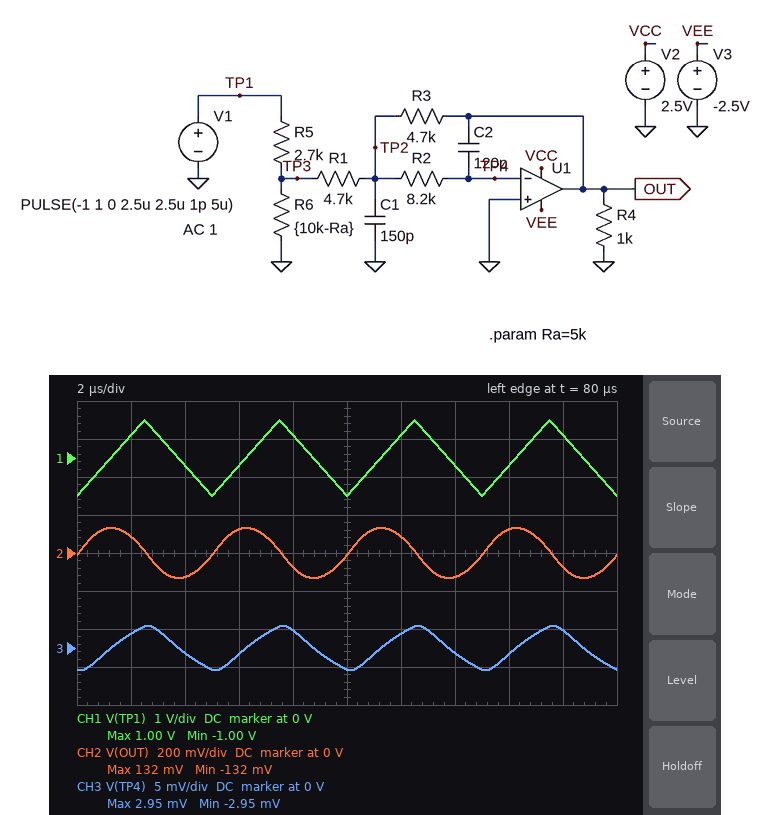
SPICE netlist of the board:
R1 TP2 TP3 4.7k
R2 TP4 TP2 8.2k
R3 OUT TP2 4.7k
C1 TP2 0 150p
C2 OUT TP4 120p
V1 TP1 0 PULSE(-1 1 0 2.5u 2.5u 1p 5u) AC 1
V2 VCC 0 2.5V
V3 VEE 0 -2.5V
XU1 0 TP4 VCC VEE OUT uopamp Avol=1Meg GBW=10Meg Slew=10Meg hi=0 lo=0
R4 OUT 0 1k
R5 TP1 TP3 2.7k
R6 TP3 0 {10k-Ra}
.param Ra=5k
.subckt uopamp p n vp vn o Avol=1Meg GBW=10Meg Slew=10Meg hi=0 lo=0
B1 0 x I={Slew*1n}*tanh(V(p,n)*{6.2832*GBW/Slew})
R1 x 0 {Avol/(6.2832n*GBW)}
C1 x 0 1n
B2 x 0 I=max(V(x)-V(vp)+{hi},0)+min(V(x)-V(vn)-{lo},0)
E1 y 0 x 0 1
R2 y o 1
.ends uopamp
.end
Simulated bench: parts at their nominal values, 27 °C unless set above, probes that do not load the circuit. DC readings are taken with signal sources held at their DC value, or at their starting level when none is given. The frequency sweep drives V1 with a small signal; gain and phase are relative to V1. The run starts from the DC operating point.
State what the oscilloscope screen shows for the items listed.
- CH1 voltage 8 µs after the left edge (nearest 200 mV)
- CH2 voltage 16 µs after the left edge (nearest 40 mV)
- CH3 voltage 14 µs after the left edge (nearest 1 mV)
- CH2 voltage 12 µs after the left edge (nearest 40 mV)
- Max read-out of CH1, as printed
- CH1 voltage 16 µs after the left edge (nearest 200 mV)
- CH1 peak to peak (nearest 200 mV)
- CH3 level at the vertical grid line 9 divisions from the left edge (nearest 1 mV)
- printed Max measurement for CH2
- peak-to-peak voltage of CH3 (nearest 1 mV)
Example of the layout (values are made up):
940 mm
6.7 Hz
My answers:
600 mV
120 mV
-1 mV
80 mV
1.00 V
-200 mV
2.0 V
2 mV
132 mV
6 mV
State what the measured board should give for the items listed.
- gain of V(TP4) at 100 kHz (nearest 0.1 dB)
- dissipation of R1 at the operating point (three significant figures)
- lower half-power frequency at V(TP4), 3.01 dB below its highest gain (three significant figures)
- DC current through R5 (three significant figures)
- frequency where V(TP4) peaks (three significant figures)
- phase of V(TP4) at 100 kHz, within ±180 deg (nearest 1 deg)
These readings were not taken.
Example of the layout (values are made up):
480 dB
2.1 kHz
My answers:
-50.6 dB
47.6 µW
62.3 kHz
195 µA
189 kHz
26 deg
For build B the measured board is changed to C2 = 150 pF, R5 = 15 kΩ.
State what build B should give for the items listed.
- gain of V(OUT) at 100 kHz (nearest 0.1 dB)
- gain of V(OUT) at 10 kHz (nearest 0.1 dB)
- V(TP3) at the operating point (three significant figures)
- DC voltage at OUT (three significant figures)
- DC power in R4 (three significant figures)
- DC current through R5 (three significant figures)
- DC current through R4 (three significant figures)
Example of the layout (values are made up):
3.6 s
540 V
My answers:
-22.1 dB
-17.2 dB
-139 mV
139 mV
19.3 µW
57.4 µA
139 µA
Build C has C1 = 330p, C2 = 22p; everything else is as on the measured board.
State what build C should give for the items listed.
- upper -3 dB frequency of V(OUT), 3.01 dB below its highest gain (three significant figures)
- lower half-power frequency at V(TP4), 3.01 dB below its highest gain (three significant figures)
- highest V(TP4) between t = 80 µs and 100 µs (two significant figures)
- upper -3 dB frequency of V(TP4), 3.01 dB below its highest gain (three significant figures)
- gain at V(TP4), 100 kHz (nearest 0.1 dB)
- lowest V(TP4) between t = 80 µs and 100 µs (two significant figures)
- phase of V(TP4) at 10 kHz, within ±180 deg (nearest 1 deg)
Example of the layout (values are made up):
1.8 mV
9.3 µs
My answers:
343 kHz
197 kHz
9.8 mV
421 kHz
-45.8 dB
-9.8 mV
88 deg
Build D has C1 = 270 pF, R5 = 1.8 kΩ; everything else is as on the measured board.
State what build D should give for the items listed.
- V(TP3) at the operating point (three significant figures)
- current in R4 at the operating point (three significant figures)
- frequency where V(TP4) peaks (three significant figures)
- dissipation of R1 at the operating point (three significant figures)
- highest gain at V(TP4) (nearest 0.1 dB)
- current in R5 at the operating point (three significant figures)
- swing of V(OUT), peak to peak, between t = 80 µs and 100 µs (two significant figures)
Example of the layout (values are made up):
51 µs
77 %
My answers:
-574 mV
574 µA
141 kHz
70.0 µW
-48.1 dB
237 µA
300 mV
